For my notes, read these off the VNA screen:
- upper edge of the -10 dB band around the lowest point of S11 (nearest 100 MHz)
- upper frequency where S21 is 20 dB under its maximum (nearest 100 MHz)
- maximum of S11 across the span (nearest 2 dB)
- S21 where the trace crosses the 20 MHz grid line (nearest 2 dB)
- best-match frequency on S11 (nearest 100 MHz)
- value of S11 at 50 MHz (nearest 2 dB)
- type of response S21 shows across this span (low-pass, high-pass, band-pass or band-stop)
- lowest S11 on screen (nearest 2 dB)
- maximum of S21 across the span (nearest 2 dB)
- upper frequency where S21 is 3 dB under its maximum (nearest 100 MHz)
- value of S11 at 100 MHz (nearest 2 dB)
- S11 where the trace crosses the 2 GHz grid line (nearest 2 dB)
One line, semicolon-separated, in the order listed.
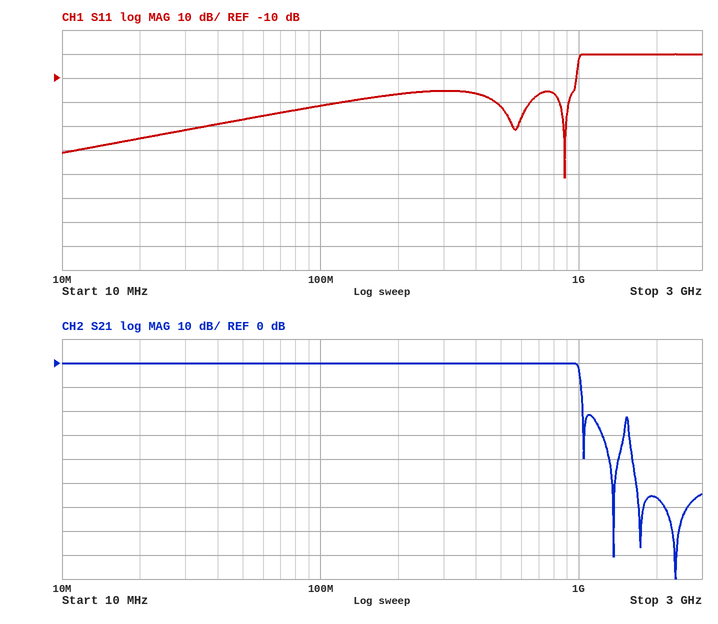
1.0 GHz; 1.0 GHz; 0 dB; 0 dB; 900 MHz; -28 dB; low-pass; -52 dB; 0 dB; 1.0 GHz; -22 dB; 0 dB
